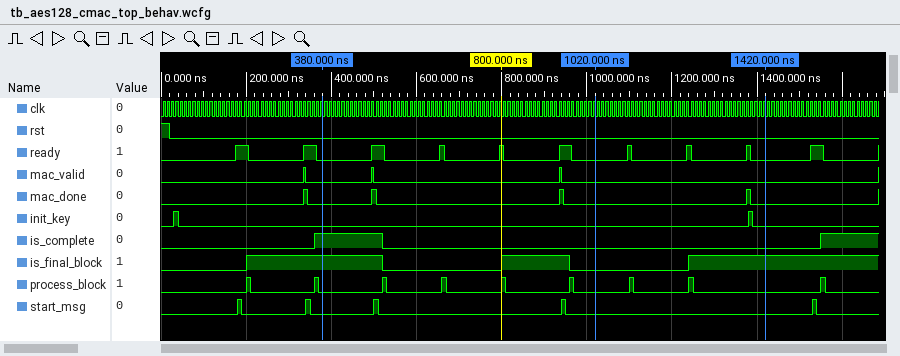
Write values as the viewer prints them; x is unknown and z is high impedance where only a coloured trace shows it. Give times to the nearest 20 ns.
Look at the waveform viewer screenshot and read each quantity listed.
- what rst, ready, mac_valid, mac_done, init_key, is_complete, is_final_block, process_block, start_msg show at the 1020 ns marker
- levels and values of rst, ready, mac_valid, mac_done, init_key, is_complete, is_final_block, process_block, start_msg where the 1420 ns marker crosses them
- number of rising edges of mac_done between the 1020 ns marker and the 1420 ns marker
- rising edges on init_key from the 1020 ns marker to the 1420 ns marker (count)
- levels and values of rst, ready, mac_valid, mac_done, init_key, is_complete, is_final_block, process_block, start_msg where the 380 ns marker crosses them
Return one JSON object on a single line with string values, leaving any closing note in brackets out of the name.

{"what rst, ready, mac_valid, mac_done, init_key, is_complete, is_final_block, process_block, start_msg show at the 1020 ns marker": "rst=0, ready=0, mac_valid=0, mac_done=0, init_key=0, is_complete=0, is_final_block=0, process_block=0, start_msg=0", "levels and values of rst, ready, mac_valid, mac_done, init_key, is_complete, is_final_block, process_block, start_msg where the 1420 ns marker crosses them": "rst=0, ready=0, mac_valid=0, mac_done=0, init_key=0, is_complete=0, is_final_block=1, process_block=0, start_msg=0", "number of rising edges of mac_done between the 1020 ns marker and the 1420 ns marker": "1", "rising edges on init_key from the 1020 ns marker to the 1420 ns marker": "1", "levels and values of rst, ready, mac_valid, mac_done, init_key, is_complete, is_final_block, process_block, start_msg where the 380 ns marker crosses them": "rst=0, ready=0, mac_valid=0, mac_done=0, init_key=0, is_complete=1, is_final_block=1, process_block=0, start_msg=0"}
